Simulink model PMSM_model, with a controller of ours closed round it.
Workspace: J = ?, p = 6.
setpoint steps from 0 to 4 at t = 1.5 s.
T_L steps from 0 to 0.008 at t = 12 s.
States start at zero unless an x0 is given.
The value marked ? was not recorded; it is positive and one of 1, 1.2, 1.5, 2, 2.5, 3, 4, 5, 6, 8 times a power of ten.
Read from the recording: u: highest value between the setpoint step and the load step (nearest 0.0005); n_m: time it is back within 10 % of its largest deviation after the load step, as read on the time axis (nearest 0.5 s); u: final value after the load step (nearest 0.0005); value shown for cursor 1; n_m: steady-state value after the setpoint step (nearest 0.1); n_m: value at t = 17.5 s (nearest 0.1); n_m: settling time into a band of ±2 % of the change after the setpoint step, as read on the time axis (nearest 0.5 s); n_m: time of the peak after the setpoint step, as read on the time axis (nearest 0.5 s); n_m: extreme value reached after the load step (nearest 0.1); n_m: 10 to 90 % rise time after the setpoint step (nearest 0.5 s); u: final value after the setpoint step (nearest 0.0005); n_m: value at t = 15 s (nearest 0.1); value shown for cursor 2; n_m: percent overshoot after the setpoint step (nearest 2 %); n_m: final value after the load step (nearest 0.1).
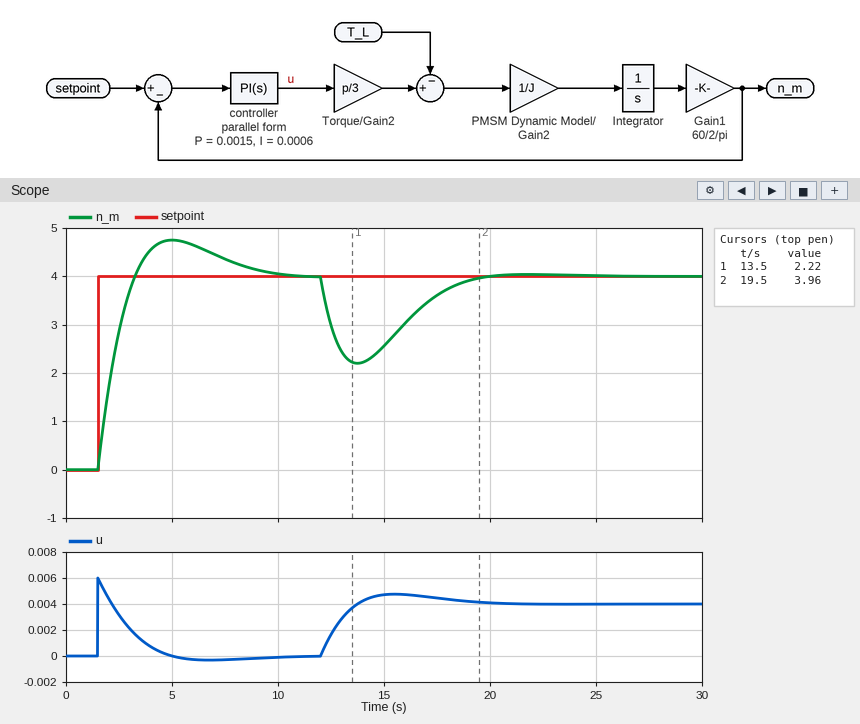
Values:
0.0060
18.5 s
0.0040
2.22
4.0
3.6
9.5 s
5.0 s
2.2
1.5 s
0.0000
2.6
3.96
18 %
4.0
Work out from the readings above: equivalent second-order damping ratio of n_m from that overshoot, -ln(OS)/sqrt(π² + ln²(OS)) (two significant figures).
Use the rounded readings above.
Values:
0.48
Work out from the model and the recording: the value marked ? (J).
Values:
0.03
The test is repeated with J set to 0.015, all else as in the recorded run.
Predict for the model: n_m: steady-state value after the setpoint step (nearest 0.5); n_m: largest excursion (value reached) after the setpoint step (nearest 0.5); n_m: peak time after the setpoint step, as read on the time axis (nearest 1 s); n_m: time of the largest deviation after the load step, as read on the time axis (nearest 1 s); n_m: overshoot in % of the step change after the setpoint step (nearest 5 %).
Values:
4.0
4.5
4 s
13 s
10 %
